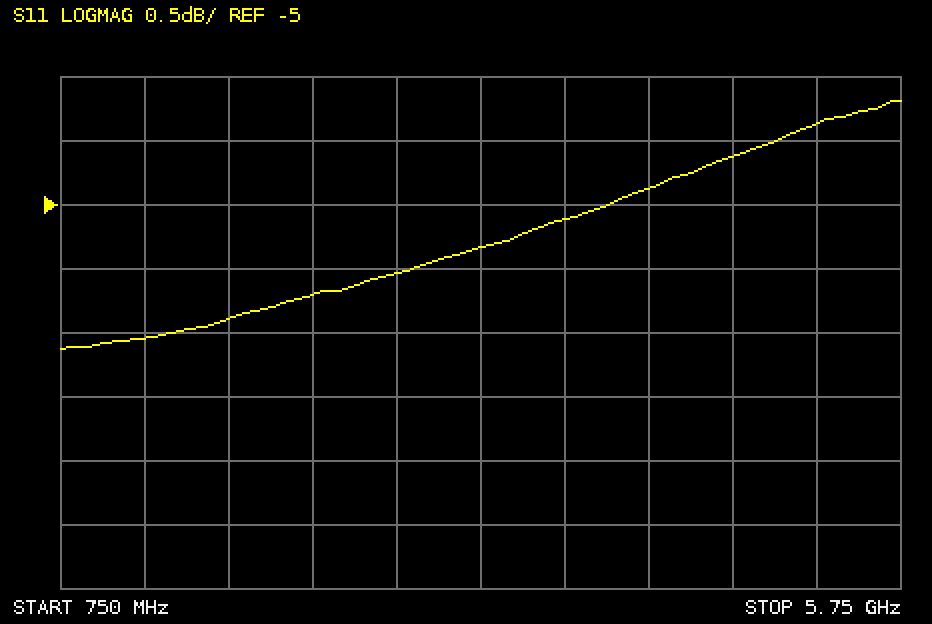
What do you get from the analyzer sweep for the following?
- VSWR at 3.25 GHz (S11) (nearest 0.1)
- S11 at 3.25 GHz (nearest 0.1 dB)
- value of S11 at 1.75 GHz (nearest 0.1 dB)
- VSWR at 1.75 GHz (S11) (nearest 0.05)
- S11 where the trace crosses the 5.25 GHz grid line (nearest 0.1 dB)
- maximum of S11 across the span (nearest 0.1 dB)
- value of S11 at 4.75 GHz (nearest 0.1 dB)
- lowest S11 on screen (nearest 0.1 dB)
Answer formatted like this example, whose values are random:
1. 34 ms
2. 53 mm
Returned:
1. 3.4
2. -5.3 dB
3. -5.9 dB
4. 3.05
5. -4.4 dB
6. -4.2 dB
7. -4.6 dB
8. -6.1 dB
